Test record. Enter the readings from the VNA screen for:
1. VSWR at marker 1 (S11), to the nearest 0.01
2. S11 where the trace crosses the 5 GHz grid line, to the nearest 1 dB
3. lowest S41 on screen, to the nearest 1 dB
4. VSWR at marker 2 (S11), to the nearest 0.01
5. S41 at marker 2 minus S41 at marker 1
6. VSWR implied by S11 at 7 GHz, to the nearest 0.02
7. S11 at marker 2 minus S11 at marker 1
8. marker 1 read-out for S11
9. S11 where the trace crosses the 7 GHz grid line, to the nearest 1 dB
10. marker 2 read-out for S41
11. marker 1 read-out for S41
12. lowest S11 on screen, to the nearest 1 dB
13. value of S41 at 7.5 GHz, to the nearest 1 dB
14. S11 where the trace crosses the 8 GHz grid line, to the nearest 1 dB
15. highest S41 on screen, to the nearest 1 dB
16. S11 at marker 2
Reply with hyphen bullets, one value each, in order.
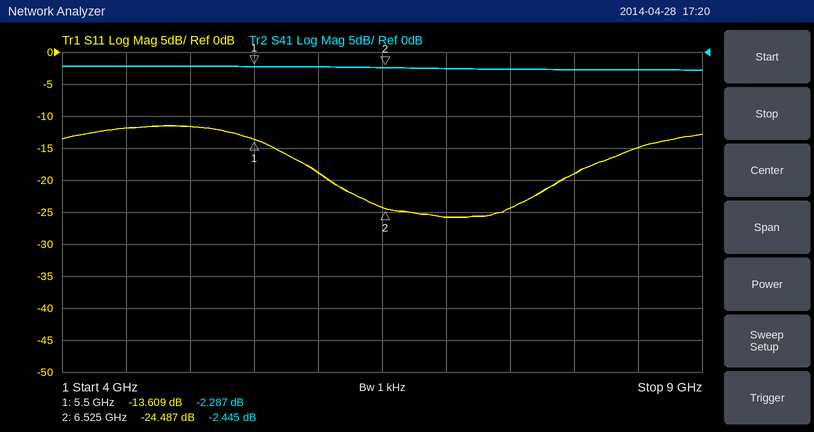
- 1.53
- -12 dB
- -3 dB
- 1.13
- -0.158 dB
- 1.10
- -10.878 dB
- -13.609 dB
- -26 dB
- -2.445 dB
- -2.287 dB
- -26 dB
- -3 dB
- -19 dB
- -2 dB
- -24.487 dB
